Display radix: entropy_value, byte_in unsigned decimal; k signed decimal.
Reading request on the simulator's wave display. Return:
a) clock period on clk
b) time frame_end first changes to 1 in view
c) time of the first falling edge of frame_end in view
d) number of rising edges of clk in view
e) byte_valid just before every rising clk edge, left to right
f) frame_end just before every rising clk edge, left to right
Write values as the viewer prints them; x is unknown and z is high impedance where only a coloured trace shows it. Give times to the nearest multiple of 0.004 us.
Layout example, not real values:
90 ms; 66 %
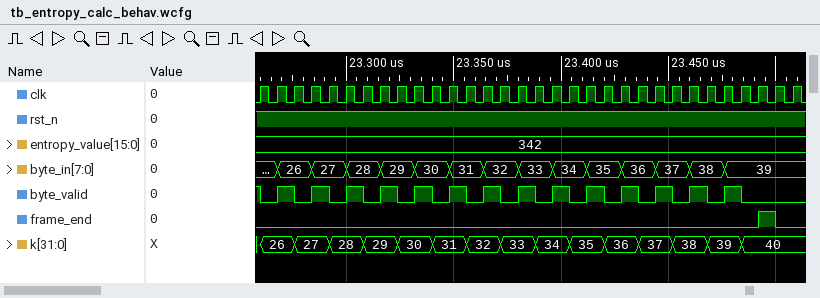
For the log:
0.008 us; 23.492 us; 23.5 us; 32; 1 0 1 0 1 0 1 0 1 0 1 0 1 0 1 0 1 0 1 0 1 0 1 0 1 0 1 0 1 0 0 0; 0 0 0 0 0 0 0 0 0 0 0 0 0 0 0 0 0 0 0 0 0 0 0 0 0 0 0 0 0 0 1 0
